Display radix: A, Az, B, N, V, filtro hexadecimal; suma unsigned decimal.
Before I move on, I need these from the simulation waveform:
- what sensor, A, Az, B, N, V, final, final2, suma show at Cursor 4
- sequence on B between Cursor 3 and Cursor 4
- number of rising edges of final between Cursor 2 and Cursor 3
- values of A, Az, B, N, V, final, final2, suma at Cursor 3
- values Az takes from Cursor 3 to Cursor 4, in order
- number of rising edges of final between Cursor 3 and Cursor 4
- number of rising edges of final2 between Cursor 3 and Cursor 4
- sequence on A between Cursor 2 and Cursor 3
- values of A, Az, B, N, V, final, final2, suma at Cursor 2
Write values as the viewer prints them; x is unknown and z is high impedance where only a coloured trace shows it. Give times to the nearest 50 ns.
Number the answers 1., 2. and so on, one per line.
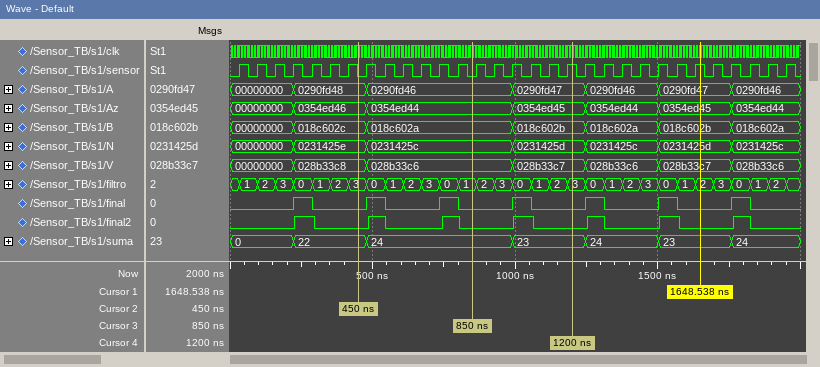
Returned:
1. sensor=1, A=0290fd47, Az=0354ed45, B=018c602b, N=0231425d, V=028b33c7, final=0, final2=0, suma=23
2. 018c602a, 018c602b
3. 2
4. A=0290fd46, Az=0354ed44, B=018c602a, N=0231425c, V=028b33c6, final=0, final2=0, suma=24
5. 0354ed44, 0354ed45
6. 1
7. 1
8. 0290fd48, 0290fd46
9. A=0290fd48, Az=0354ed46, B=018c602c, N=0231425e, V=028b33c8, final=0, final2=0, suma=22
